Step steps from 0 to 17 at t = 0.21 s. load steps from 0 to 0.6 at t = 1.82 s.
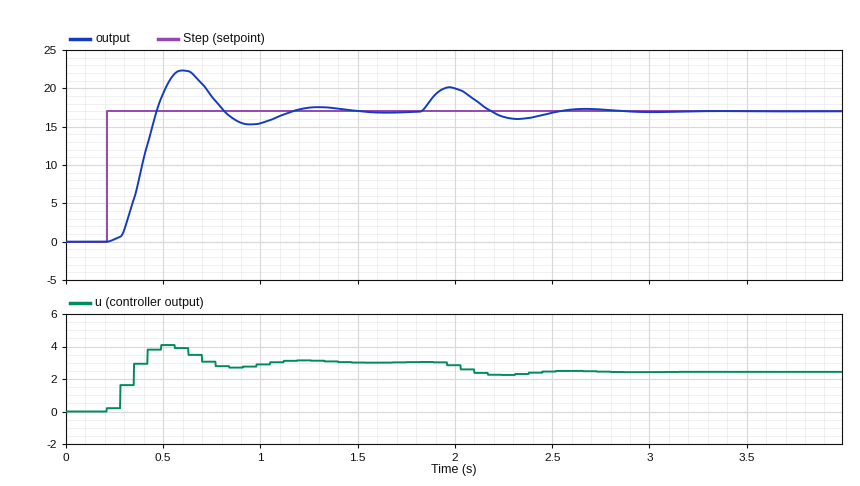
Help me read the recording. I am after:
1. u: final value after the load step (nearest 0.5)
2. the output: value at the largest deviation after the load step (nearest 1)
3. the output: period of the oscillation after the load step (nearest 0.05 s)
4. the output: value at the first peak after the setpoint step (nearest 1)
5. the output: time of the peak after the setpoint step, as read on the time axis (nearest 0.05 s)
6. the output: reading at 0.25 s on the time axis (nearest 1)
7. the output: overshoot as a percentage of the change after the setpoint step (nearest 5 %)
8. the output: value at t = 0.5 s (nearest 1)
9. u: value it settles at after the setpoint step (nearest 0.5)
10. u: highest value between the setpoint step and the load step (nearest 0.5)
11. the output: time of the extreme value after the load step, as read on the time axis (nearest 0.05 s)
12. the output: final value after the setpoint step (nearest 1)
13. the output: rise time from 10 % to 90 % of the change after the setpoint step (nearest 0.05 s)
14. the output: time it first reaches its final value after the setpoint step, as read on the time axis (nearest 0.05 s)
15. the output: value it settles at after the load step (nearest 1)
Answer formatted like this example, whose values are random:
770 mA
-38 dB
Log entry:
2.5
20
0.70 s
22
0.60 s
0
30 %
19
3.0
4.0
1.95 s
17
0.15 s
0.45 s
17
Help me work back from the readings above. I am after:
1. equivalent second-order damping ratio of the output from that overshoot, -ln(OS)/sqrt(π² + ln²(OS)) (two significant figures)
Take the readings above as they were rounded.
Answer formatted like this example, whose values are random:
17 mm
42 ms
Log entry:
0.36
